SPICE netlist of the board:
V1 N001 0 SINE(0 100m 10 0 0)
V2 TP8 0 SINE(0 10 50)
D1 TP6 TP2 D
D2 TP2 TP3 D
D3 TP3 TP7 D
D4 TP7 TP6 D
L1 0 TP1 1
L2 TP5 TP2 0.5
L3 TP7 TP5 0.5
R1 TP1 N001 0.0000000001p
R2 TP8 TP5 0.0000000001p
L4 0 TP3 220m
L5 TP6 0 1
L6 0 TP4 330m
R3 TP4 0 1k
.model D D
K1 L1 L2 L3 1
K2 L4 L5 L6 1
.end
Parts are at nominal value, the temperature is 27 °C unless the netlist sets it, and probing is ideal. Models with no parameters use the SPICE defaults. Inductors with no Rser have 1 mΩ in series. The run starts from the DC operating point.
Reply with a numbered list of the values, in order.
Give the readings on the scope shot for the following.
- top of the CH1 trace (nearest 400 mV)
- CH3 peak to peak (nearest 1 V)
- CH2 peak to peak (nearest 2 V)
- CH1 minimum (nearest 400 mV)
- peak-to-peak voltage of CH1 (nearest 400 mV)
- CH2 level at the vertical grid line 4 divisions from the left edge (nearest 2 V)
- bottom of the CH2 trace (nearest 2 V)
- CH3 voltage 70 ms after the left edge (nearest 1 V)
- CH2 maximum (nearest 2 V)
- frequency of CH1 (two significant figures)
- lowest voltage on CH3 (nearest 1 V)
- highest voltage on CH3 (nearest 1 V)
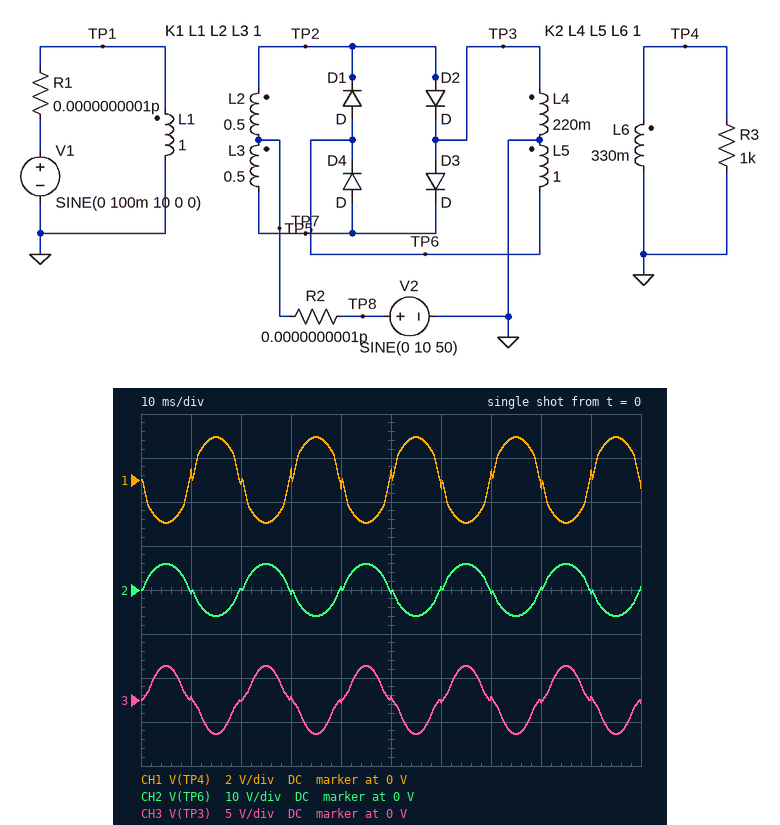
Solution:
1. 2.0 V
2. 8 V
3. 12 V
4. -2.0 V
5. 4.0 V
6. 0 V
7. -6 V
8. 0 V
9. 6 V
10. 50 Hz
11. -4 V
12. 4 V
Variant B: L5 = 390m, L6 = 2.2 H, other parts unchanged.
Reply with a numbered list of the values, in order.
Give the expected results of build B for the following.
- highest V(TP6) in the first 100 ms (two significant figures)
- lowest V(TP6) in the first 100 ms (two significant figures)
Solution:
1. 5.6 V
2. -5.6 V
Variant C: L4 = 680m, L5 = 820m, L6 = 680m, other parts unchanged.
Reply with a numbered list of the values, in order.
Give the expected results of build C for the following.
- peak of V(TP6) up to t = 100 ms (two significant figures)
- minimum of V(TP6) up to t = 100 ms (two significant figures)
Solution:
1. 5.0 V
2. -5.0 V
